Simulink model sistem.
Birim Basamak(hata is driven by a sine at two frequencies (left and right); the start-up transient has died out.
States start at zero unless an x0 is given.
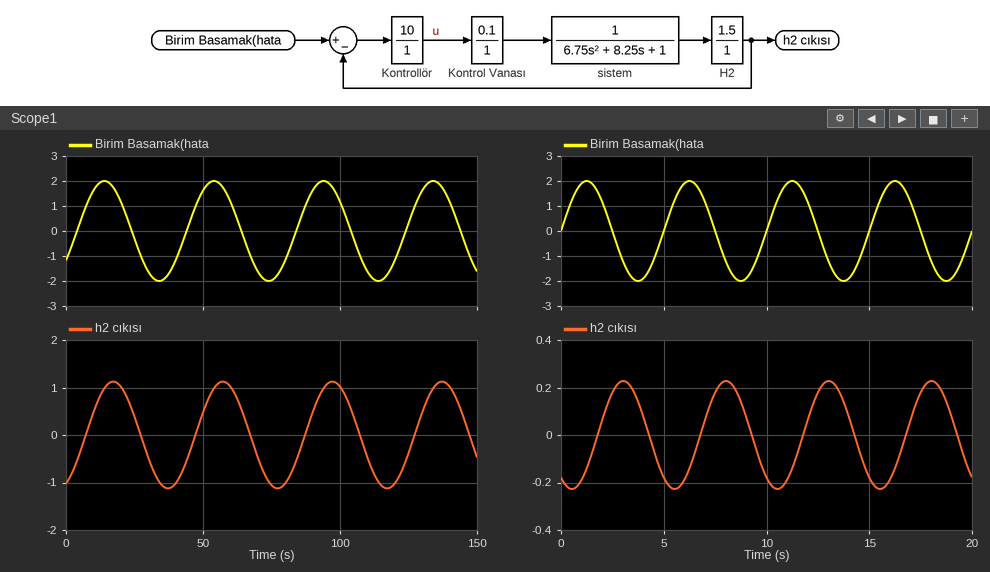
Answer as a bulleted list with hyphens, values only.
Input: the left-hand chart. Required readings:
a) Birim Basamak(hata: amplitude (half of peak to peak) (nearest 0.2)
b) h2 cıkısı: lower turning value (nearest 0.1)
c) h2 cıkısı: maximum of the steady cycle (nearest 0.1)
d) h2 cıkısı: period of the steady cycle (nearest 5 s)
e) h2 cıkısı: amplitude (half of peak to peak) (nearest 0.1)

- 2.0
- -1.1
- 1.1
- 40 s
- 1.1
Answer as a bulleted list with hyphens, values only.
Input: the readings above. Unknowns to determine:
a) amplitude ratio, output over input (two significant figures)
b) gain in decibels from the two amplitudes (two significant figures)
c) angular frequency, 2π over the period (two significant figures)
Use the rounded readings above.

- 0.55
- -5.2 dB
- 0.16 rad/s
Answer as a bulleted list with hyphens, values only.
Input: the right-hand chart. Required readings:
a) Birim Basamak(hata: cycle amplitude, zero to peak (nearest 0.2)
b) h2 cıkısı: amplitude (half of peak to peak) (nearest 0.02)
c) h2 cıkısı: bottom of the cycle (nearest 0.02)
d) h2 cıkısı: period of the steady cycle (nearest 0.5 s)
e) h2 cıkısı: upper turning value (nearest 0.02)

- 2.0
- 0.22
- -0.22
- 5.0 s
- 0.22
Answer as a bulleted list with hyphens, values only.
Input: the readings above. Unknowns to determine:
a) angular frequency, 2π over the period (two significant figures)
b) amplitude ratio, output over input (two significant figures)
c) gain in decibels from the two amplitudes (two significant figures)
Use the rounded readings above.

- 1.3 rad/s
- 0.11
- -19 dB
